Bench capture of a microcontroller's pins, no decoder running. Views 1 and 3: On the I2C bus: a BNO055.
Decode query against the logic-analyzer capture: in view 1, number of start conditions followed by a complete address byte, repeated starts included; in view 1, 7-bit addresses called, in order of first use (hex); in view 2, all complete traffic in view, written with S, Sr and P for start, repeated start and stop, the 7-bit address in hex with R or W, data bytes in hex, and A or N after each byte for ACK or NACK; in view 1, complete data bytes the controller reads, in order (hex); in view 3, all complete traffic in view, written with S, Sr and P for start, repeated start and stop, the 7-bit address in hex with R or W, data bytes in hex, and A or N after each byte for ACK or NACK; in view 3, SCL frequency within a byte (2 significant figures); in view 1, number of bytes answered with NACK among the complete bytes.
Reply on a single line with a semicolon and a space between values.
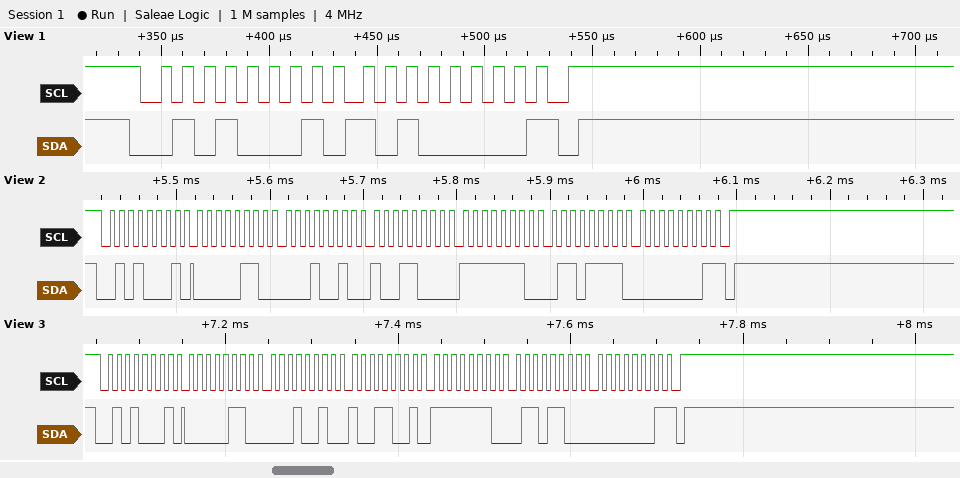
1; 0x28; S 28R A 06 A 12 A 98 A FE A 6F A 01 N P; A0; S 28R A 06 A 12 A 99 A FE A 6C A 01 N P; 100 kHz; 1
